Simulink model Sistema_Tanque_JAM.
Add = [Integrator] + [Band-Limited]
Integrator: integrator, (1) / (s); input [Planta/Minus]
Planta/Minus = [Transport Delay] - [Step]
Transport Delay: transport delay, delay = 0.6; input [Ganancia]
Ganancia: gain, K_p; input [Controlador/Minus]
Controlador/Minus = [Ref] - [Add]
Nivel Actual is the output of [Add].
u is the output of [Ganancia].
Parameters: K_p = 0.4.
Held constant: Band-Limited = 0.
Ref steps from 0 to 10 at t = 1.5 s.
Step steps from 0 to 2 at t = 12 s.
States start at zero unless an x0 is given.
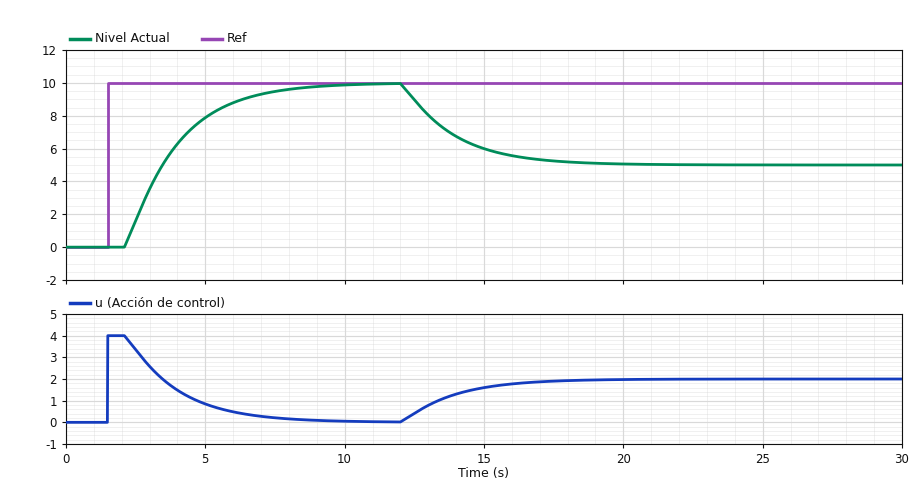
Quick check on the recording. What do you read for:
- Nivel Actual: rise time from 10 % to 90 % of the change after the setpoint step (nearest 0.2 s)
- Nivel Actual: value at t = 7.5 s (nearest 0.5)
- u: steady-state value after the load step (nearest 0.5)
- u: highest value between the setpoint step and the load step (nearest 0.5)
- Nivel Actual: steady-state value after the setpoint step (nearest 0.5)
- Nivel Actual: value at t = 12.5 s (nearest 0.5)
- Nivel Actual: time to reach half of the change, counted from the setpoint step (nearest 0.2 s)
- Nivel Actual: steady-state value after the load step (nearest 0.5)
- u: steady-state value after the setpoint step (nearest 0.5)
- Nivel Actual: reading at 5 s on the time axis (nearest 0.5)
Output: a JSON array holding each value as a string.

["4.0 s", "9.5", "2.0", "4.0", "10.0", "9.0", "2.0 s", "5.0", "0.0", "8.0"]
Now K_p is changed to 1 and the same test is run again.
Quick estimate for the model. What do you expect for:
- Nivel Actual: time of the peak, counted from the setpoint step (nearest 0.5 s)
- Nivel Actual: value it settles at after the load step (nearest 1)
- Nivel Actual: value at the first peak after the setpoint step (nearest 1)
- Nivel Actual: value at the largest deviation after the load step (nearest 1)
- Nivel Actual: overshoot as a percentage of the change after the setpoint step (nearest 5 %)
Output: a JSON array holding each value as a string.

["2.5 s", "8", "11", "8", "10 %"]
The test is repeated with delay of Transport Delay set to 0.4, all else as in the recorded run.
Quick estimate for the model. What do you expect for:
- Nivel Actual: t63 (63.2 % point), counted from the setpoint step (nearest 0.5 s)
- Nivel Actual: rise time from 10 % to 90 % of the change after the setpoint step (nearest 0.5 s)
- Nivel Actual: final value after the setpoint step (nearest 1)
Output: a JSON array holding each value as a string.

["2.5 s", "4.5 s", "10"]
